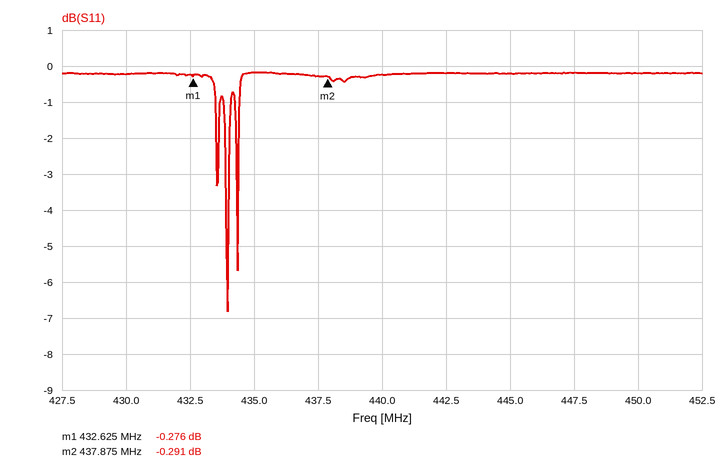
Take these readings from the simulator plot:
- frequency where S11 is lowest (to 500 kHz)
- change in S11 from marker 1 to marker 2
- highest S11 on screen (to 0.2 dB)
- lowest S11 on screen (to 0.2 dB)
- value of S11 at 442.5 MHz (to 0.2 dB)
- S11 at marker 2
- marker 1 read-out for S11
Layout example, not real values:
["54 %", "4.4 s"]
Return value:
["434.0 MHz", "-0.015 dB", "-0.2 dB", "-6.8 dB", "-0.2 dB", "-0.291 dB", "-0.276 dB"]
